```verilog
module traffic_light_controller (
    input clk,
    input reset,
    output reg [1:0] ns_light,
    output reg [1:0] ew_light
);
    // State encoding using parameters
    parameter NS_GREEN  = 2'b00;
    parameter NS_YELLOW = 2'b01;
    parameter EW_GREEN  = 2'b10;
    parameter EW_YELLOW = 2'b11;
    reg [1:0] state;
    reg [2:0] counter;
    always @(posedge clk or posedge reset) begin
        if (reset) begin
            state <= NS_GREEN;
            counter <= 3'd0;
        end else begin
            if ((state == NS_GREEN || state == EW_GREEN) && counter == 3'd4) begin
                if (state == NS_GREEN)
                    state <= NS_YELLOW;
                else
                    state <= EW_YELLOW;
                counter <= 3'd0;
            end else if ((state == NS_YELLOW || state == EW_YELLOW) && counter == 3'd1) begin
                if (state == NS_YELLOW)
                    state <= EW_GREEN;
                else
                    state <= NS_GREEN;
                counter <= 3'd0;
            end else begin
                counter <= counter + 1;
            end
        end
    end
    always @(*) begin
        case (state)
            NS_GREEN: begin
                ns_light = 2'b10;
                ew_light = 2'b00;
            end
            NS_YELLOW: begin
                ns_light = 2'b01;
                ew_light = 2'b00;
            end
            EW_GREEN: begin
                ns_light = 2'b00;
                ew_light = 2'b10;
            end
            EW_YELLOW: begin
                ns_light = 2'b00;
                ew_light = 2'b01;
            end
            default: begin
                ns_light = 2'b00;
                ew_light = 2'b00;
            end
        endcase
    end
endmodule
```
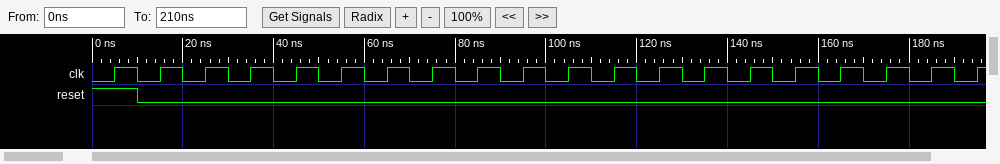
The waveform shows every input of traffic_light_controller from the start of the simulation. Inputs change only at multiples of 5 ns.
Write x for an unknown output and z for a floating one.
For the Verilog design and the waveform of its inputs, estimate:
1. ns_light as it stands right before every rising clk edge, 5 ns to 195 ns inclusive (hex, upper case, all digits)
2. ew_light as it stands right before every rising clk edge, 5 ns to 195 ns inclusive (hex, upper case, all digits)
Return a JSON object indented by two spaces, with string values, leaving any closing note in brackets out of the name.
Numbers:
{
  "ns_light as it stands right before every rising clk edge, 5 ns to 195 ns inclusive": "2, 2, 2, 2, 2, 2, 1, 1, 0, 0, 0, 0, 0, 0, 0, 2, 2, 2, 2, 2",
  "ew_light as it stands right before every rising clk edge, 5 ns to 195 ns inclusive": "0, 0, 0, 0, 0, 0, 0, 0, 2, 2, 2, 2, 2, 1, 1, 0, 0, 0, 0, 0"
}
